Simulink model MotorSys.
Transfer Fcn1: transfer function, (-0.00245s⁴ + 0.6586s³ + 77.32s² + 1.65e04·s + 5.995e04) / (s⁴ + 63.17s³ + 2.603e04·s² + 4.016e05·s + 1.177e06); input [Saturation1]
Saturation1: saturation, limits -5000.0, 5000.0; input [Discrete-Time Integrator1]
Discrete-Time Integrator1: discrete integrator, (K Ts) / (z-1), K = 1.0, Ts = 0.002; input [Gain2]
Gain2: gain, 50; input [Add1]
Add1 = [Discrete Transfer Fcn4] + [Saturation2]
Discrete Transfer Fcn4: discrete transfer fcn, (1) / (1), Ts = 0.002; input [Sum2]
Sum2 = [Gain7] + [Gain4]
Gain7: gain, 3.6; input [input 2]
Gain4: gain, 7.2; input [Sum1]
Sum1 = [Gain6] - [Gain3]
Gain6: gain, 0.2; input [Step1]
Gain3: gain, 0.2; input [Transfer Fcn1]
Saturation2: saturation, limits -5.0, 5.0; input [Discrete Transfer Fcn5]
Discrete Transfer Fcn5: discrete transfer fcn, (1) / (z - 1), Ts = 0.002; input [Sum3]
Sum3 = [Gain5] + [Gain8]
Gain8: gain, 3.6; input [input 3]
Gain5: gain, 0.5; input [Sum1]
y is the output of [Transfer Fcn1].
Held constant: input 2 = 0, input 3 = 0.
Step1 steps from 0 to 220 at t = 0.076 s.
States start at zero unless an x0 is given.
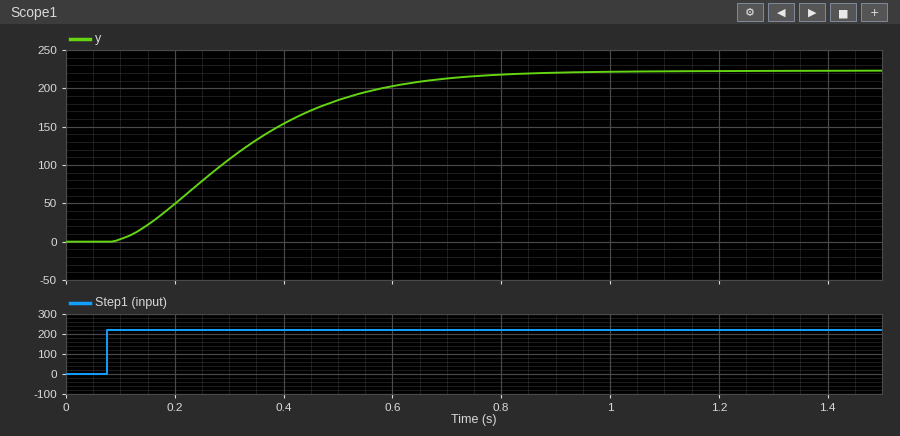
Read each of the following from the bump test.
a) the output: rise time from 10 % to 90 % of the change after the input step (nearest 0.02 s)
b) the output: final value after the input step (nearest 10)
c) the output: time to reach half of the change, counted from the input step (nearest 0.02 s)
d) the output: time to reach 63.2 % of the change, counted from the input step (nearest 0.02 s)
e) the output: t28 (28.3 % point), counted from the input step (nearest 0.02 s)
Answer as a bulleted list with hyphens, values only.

- 0.44 s
- 220
- 0.24 s
- 0.30 s
- 0.14 s
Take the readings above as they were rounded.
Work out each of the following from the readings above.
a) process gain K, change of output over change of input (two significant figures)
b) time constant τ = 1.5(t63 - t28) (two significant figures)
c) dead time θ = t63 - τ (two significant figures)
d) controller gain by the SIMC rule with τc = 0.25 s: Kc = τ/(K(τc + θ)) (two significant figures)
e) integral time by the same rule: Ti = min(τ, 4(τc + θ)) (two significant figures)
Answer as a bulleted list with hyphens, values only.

- 1.0
- 0.24 s
- 0.060 s
- 0.77
- 0.24 s
